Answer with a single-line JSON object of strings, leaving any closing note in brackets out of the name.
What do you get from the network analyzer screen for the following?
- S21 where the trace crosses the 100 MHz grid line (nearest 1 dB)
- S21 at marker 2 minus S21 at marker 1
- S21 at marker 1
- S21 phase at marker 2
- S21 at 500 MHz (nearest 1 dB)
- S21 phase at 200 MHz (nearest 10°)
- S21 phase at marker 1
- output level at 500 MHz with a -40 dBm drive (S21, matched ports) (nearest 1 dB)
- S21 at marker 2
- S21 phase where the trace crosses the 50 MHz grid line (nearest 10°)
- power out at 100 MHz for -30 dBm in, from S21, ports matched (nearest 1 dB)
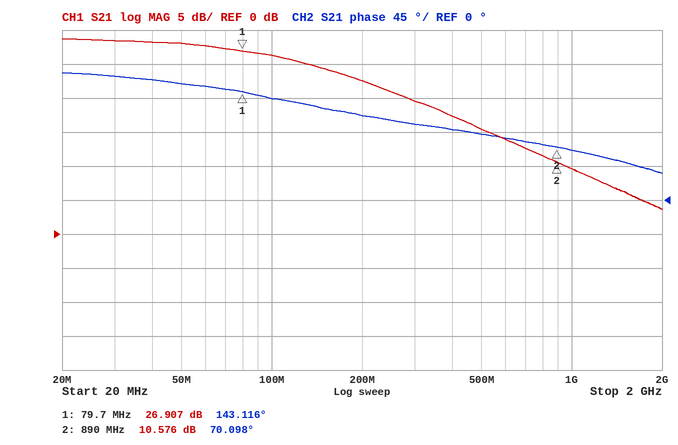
{"S21 where the trace crosses the 100 MHz grid line": "26 dB", "S21 at marker 2 minus S21 at marker 1": "-16.331 dB", "S21 at marker 1": "26.907 dB", "S21 phase at marker 2": "70.098°", "S21 at 500 MHz": "15 dB", "S21 phase at 200 MHz": "110°", "S21 phase at marker 1": "143.116°", "output level at 500 MHz with a -40 dBm drive (S21, matched ports)": "-25 dBm", "S21 at marker 2": "10.576 dB", "S21 phase where the trace crosses the 50 MHz grid line": "150°", "power out at 100 MHz for -30 dBm in, from S21, ports matched": "-4 dBm"}
